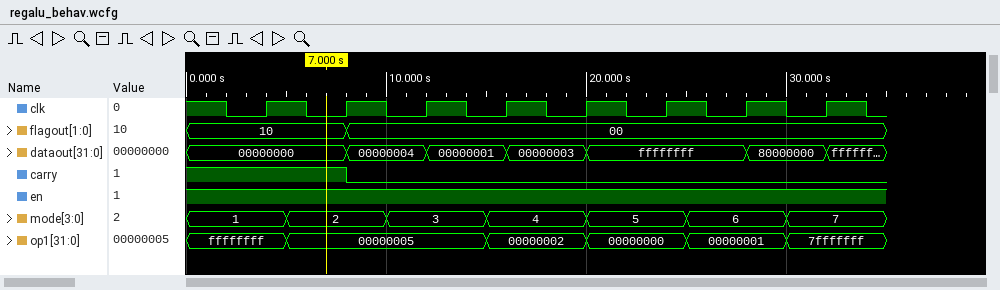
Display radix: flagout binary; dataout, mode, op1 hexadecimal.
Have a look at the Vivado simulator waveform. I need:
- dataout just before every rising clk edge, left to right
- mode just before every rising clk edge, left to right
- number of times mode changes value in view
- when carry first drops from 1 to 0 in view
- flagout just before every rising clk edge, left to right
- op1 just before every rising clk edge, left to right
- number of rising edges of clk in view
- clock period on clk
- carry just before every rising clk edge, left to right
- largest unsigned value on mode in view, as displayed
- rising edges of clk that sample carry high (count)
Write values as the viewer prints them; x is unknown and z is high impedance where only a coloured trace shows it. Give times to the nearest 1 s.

00000000, 00000000, 00000004, 00000001, 00000003, ffffffff, ffffffff, 80000000
1, 2, 3, 4, 4, 5, 6, 7
6
8 s
10, 10, 00, 00, 00, 00, 00, 00
ffffffff, 00000005, 00000005, 00000002, 00000002, 00000000, 00000001, 7fffffff
8
4 s
1 1 0 0 0 0 0 0
7
2
